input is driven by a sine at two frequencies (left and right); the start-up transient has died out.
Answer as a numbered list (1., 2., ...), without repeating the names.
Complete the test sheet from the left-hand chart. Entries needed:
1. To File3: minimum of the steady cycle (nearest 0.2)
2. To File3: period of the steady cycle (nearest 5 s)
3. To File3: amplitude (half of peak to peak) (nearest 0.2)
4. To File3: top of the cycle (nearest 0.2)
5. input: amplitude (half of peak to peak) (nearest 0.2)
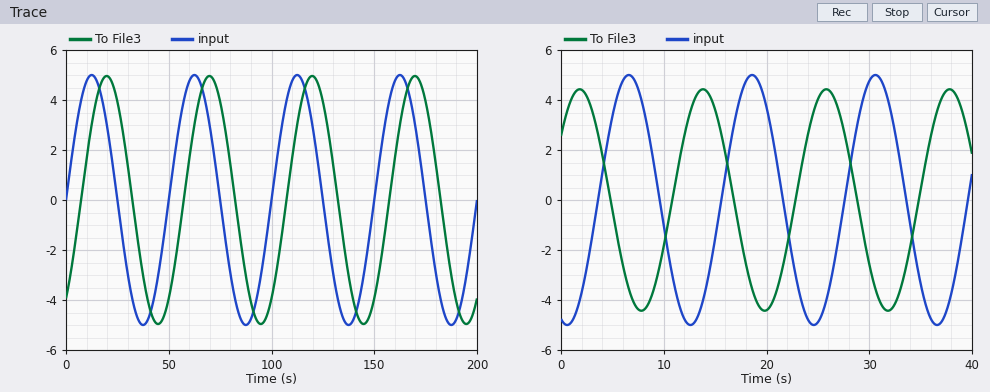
1. -5.0
2. 50 s
3. 5.0
4. 5.0
5. 5.0
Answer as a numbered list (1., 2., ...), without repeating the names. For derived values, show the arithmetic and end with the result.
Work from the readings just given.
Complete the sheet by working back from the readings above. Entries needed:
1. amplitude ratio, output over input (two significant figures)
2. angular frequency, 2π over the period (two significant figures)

1. 5 / 5 = 1.0
2. 2π / 50 = 0.13 rad/s
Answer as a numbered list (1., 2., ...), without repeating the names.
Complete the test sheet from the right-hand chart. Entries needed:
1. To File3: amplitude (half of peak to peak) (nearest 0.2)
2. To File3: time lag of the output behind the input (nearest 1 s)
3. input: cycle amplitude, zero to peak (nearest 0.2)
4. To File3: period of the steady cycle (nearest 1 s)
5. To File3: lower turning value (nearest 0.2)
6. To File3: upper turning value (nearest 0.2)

1. 4.4
2. 7 s
3. 5.0
4. 12 s
5. -4.4
6. 4.4
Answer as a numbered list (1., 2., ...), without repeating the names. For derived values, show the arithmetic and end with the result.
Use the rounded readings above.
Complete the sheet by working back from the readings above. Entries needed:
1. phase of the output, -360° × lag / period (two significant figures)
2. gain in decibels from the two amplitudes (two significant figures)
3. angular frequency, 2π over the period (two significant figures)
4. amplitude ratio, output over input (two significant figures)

1. -360 × 7 / 12 = -210°
2. 20 log10(4.4 / 5) = -1.1 dB
3. 2π / 12 = 0.52 rad/s
4. 4.4 / 5 = 0.88
